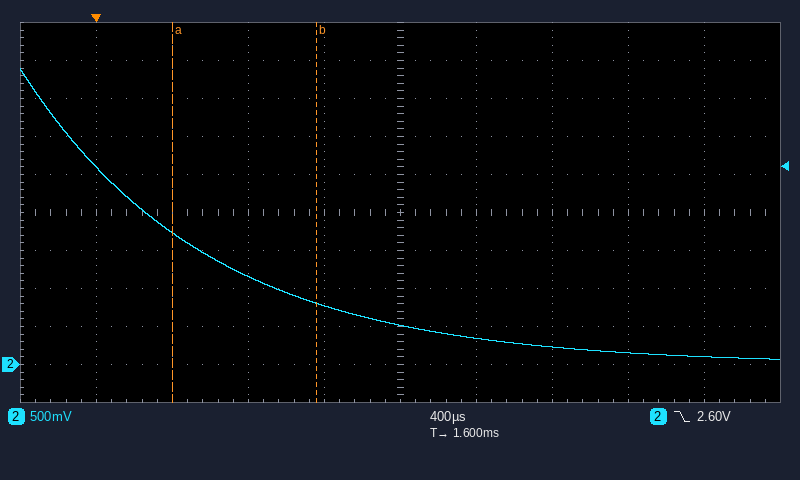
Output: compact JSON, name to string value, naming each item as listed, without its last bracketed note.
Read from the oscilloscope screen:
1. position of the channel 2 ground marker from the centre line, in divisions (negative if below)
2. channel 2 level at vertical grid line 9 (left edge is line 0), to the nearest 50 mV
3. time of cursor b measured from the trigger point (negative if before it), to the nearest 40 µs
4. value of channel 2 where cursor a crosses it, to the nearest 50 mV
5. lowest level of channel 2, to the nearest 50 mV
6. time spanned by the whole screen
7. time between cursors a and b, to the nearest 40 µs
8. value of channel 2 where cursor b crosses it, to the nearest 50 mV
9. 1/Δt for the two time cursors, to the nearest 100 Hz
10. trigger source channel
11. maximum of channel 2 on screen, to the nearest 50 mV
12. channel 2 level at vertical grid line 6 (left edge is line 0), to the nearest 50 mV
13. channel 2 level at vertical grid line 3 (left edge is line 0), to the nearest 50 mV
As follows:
{"position of the channel 2 ground marker from the centre line, in divisions": "-4.0 div", "channel 2 level at vertical grid line 9 (left edge is line 0), to the nearest 50 mV": "100 mV", "time of cursor b measured from the trigger point (negative if before it), to the nearest 40 µs": "+1.16 ms", "value of channel 2 where cursor a crosses it, to the nearest 50 mV": "1.75 V", "lowest level of channel 2, to the nearest 50 mV": "50 mV", "time spanned by the whole screen": "4 ms", "time between cursors a and b, to the nearest 40 µs": "760 µs", "value of channel 2 where cursor b crosses it, to the nearest 50 mV": "800 mV", "1/Δt for the two time cursors, to the nearest 100 Hz": "1.3 kHz", "trigger source channel": "channel 2", "maximum of channel 2 on screen, to the nearest 50 mV": "3.90 V", "channel 2 level at vertical grid line 6 (left edge is line 0), to the nearest 50 mV": "350 mV", "channel 2 level at vertical grid line 3 (left edge is line 0), to the nearest 50 mV": "1.15 V"}
